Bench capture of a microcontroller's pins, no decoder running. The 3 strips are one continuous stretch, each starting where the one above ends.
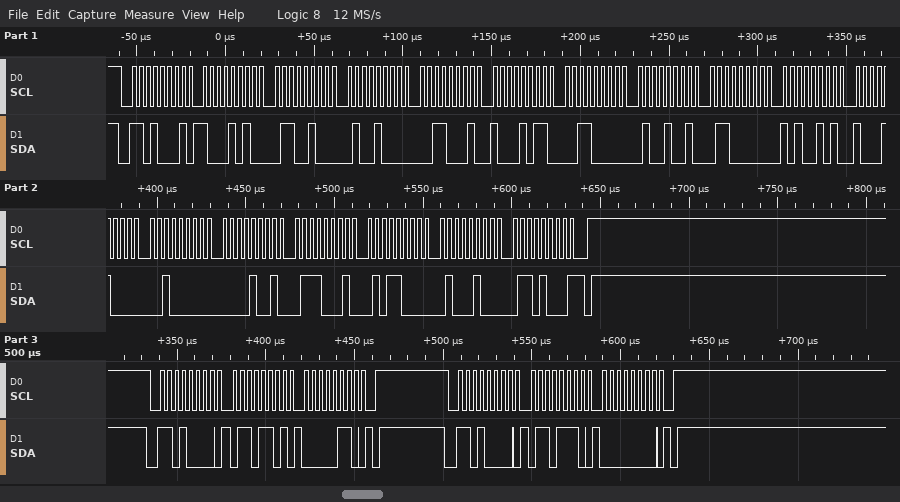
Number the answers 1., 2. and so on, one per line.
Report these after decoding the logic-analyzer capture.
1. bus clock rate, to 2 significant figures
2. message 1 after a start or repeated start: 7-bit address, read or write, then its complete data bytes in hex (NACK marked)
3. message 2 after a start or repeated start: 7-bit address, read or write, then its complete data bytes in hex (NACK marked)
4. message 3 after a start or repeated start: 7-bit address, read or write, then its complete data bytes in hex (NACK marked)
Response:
1. 250 kHz
2. 0x68 read: 8A 64 48 31 8B 30 49 60 A5 88 20 09 71 58 44 68 NACK
3. 0x68 write: 6D 06
4. 0x68 write: 6E 00
